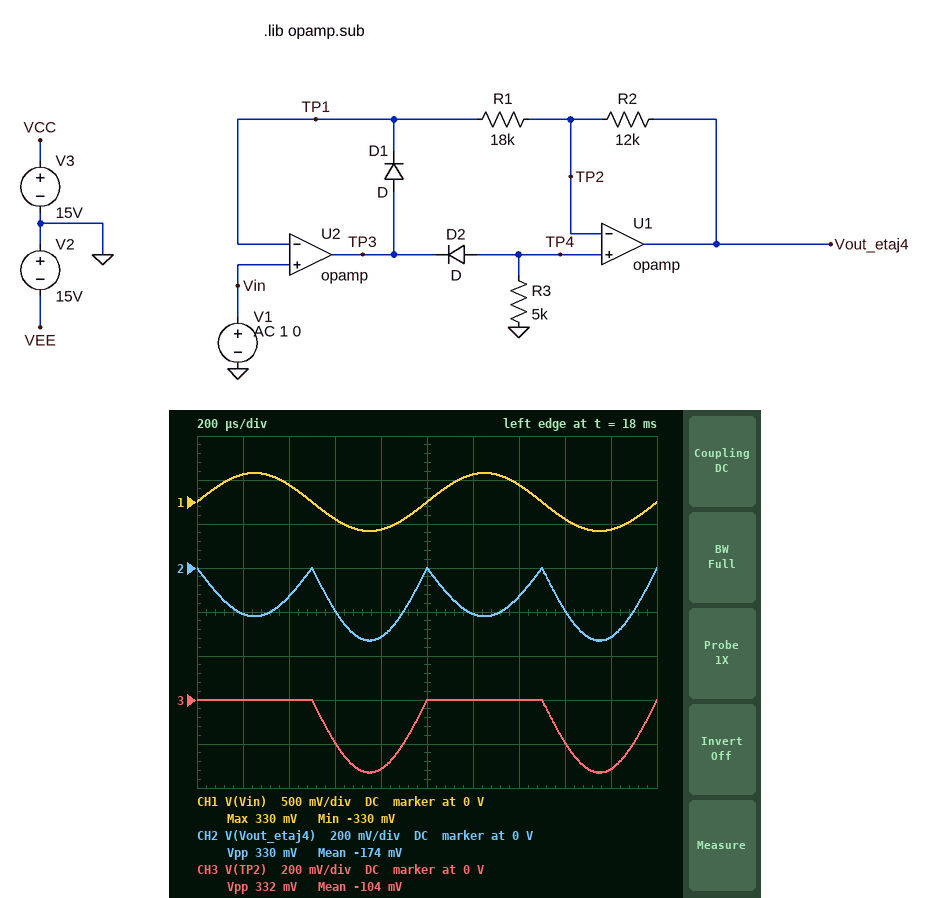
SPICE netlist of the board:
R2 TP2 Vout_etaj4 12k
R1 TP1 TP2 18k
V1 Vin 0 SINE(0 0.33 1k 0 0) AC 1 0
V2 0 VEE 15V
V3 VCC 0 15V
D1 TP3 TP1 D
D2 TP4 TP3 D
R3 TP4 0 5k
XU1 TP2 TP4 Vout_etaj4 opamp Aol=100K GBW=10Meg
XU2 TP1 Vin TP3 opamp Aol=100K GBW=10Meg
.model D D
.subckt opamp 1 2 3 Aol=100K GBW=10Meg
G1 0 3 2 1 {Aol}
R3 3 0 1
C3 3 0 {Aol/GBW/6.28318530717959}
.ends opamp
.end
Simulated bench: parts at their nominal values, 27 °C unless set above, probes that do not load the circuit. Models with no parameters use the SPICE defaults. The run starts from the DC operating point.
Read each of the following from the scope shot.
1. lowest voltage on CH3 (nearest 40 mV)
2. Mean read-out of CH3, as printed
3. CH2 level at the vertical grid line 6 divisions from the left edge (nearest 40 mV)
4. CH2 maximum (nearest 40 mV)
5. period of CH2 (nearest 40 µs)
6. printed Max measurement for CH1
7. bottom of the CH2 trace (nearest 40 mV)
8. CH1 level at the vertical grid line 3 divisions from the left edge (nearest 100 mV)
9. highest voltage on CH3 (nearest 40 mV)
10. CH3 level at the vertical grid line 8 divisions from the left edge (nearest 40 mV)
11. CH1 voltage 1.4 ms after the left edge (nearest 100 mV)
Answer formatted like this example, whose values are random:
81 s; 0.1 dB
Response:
-320 mV; -104 mV; -200 mV; 0 V; 1.00 ms; 330 mV; -320 mV; -200 mV; 0 V; -200 mV; 200 mV
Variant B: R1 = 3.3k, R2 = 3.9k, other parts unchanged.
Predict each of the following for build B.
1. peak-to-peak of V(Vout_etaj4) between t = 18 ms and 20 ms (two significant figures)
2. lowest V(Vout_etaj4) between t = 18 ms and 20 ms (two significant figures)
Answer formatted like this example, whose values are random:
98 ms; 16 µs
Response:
390 mV; -390 mV
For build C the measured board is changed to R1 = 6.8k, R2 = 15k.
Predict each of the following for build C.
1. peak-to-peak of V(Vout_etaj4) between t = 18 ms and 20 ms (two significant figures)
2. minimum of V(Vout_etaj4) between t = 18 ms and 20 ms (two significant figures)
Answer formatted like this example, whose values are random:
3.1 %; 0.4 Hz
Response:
730 mV; -730 mV
